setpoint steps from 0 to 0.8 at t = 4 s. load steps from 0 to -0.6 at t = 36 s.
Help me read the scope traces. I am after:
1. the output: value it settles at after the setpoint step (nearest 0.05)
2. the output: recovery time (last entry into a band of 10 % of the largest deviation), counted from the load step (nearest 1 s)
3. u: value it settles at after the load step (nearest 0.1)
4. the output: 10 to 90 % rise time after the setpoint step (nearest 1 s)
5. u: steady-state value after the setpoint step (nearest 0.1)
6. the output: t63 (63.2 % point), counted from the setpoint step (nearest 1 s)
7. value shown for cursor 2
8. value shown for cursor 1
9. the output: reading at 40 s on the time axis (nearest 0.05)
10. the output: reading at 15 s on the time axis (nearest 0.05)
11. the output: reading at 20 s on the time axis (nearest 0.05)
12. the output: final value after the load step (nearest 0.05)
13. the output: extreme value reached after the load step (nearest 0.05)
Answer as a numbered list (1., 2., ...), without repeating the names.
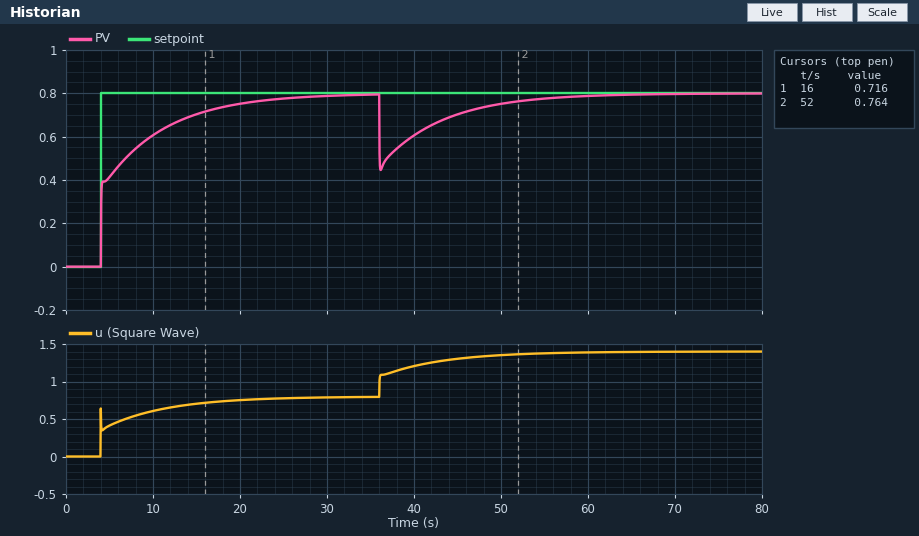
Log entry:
1. 0.80
2. 16 s
3. 1.4
4. 12 s
5. 0.8
6. 3 s
7. 0.764
8. 0.716
9. 0.60
10. 0.70
11. 0.75
12. 0.80
13. 0.45
